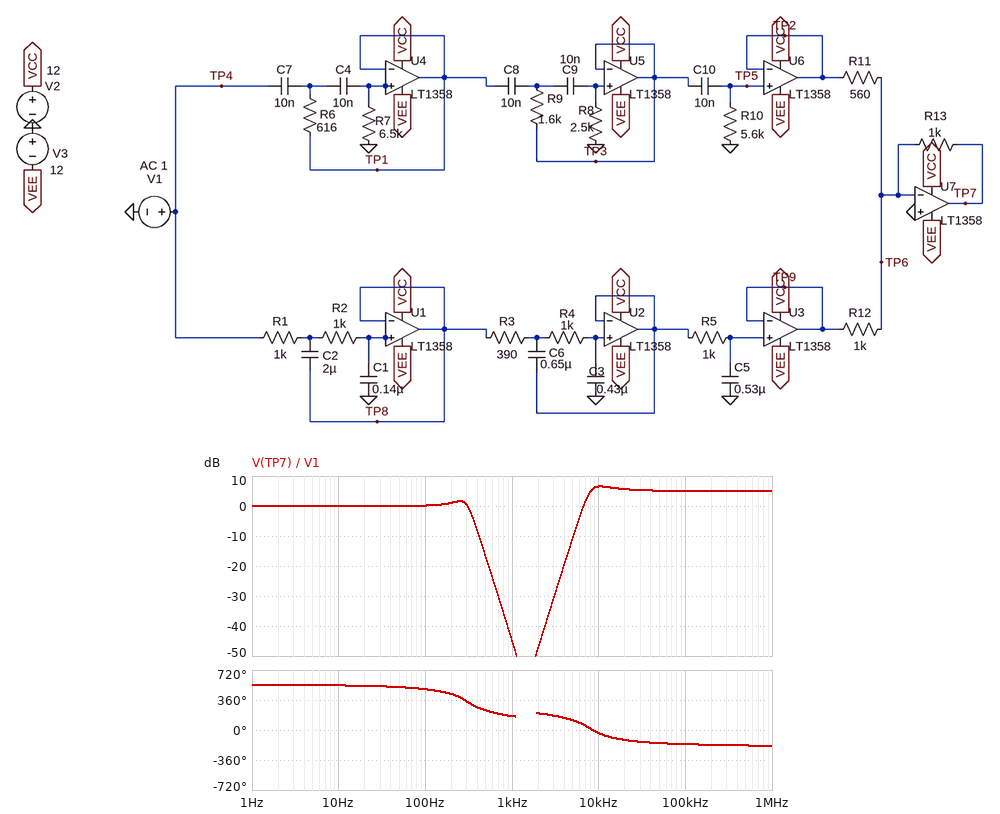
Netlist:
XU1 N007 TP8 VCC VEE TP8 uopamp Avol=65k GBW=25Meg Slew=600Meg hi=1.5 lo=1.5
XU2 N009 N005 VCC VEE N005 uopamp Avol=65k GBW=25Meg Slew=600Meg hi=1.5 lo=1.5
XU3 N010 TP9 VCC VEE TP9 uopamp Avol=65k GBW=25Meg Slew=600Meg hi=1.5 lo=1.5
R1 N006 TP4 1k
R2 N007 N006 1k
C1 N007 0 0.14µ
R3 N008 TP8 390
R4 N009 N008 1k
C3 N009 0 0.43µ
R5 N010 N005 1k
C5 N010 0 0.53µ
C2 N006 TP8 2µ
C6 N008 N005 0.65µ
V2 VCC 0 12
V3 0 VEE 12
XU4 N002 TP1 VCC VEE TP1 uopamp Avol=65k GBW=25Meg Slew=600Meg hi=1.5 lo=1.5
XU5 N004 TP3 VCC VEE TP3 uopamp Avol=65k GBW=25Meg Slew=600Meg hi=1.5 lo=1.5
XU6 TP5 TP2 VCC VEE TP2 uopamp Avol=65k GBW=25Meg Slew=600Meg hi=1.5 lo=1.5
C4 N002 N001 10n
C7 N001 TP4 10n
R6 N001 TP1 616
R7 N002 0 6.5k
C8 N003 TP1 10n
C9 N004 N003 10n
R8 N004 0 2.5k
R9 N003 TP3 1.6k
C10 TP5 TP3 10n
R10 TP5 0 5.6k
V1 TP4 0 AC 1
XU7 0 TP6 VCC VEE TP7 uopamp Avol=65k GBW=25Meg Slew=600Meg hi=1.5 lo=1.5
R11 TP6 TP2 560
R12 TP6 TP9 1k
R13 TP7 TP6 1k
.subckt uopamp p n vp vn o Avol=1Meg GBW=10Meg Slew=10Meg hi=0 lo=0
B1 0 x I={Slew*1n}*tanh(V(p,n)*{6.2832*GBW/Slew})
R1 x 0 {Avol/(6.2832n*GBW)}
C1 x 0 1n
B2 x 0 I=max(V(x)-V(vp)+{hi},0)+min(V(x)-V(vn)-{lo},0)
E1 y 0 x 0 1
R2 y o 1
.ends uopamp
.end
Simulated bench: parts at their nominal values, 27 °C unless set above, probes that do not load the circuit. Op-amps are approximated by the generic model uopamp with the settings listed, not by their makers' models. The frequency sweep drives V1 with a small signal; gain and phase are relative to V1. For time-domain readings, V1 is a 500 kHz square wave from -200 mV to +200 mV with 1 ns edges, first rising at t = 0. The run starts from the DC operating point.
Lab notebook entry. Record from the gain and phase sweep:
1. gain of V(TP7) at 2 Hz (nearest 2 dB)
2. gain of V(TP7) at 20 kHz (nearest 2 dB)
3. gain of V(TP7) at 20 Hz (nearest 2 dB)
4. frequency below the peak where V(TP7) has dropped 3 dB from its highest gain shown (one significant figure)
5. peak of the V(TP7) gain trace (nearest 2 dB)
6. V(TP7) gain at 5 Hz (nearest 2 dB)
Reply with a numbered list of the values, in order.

1. 0 dB
2. 6 dB
3. 0 dB
4. 8 kHz
5. 6 dB
6. 0 dB
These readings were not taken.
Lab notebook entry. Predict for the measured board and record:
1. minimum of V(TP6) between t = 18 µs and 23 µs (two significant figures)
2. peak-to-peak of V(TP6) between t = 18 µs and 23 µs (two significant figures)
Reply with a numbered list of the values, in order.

1. -94 mV
2. 190 mV
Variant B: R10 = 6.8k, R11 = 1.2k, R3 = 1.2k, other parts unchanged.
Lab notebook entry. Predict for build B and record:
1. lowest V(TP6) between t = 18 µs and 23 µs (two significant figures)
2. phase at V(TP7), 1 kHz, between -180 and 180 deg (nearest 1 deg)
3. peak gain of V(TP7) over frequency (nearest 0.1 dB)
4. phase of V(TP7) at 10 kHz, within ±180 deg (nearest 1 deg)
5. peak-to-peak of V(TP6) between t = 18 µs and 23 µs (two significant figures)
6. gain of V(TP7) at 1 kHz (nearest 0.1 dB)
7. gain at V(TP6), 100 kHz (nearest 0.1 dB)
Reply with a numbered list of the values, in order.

1. -51 mV
2. 145 deg
3. 0 dB
4. -40 deg
5. 100 mV
6. -53.7 dB
7. -49.5 dB
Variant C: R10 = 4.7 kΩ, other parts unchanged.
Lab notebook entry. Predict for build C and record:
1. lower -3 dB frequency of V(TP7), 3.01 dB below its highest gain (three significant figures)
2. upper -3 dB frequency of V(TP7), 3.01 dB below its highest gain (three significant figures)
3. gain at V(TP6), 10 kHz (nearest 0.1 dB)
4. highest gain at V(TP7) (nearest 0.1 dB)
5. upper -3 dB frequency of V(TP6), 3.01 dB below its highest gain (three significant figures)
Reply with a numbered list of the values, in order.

1. 7.57 kHz
2. 3.92 MHz
3. -61.6 dB
4. 6.4 dB
5. 19.1 MHz
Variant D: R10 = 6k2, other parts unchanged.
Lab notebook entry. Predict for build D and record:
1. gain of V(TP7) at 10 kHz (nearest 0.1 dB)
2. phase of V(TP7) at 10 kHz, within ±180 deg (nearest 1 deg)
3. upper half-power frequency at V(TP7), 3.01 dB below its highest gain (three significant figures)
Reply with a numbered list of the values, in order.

1. 6.6 dB
2. -39 deg
3. 3.67 MHz
